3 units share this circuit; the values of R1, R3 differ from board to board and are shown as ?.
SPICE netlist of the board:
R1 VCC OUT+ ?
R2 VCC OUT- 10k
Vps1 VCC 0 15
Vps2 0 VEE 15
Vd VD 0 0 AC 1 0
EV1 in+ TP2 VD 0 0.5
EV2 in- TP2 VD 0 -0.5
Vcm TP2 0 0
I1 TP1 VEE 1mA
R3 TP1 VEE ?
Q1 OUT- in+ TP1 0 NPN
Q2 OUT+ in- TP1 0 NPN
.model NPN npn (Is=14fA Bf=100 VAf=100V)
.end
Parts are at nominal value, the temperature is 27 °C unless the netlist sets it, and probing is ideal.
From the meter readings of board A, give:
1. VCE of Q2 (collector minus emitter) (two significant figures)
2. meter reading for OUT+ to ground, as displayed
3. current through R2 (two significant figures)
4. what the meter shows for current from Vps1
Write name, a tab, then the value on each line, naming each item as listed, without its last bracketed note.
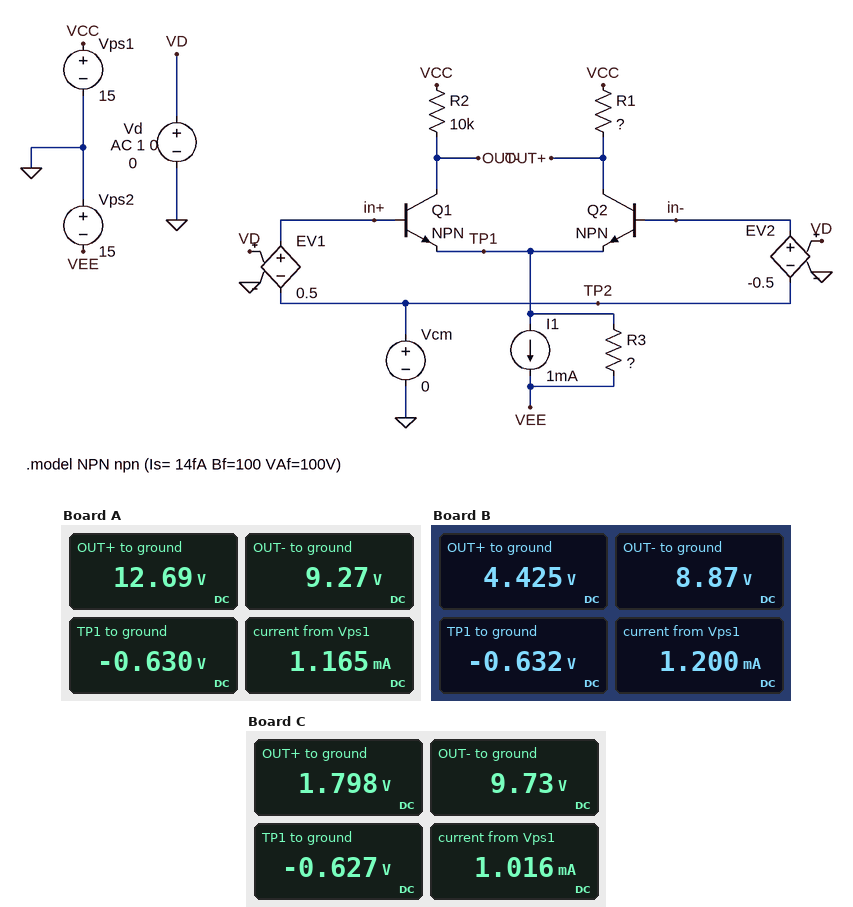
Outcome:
VCE of Q2 (collector minus emitter)	13 V
meter reading for OUT+ to ground, as displayed	12.69 V
current through R2	570 µA
what the meter shows for current from Vps1	1.165 mA
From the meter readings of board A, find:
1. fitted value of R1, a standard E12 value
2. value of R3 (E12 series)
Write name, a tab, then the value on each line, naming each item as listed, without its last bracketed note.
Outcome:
fitted value of R1, a standard E12 value	3.9 kΩ
value of R3	82 kΩ
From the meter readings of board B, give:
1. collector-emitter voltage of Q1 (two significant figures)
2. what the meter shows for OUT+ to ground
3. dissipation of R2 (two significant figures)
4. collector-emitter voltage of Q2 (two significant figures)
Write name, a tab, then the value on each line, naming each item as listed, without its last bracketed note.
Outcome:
collector-emitter voltage of Q1	9.5 V
what the meter shows for OUT+ to ground	4.425 V
dissipation of R2	3.8 mW
collector-emitter voltage of Q2	5.1 V
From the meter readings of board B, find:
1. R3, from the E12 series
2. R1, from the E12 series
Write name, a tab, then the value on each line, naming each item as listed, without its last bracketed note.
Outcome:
R3, from the E12 series	68 kΩ
R1, from the E12 series	18 kΩ
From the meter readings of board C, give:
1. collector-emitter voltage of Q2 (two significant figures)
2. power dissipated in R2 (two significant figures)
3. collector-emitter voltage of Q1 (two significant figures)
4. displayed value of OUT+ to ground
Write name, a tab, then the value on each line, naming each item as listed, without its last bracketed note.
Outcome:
collector-emitter voltage of Q2	2.4 V
power dissipated in R2	2.8 mW
collector-emitter voltage of Q1	10 V
displayed value of OUT+ to ground	1.798 V
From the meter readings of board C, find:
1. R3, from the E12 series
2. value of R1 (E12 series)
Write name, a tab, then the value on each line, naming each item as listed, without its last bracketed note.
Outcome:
R3, from the E12 series	560 kΩ
value of R1	27 kΩ
